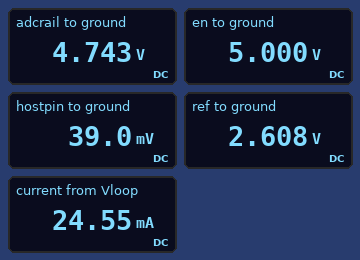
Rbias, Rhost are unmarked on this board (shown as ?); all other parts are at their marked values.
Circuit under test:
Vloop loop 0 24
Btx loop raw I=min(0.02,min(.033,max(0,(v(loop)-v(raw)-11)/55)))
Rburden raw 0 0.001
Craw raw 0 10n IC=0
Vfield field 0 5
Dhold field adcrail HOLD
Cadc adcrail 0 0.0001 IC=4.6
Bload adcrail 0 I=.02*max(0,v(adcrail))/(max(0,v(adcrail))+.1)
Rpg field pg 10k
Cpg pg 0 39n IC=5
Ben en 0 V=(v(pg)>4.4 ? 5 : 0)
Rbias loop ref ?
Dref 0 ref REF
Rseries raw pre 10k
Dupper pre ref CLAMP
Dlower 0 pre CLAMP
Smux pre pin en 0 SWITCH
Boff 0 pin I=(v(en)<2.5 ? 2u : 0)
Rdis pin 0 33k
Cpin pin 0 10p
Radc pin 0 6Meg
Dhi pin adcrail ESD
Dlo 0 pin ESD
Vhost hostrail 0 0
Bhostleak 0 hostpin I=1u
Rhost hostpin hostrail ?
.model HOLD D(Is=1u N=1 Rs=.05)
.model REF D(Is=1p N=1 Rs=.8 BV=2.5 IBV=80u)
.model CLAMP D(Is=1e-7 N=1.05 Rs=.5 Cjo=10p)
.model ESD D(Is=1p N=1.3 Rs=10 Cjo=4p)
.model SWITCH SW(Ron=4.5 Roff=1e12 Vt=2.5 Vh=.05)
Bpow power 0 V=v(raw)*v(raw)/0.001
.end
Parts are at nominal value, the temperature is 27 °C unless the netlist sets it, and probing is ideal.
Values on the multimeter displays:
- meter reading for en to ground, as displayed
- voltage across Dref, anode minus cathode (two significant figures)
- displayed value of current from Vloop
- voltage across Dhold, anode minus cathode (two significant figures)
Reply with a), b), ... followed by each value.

a) 5.000 V
b) -2.6 V
c) 24.55 mA
d) 260 mV
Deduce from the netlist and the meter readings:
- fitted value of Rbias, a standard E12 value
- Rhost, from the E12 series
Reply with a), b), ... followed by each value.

a) 4.7 kΩ
b) 39 kΩ
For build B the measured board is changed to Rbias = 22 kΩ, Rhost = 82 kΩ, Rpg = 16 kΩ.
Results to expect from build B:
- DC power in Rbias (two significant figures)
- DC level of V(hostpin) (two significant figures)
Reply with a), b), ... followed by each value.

a) 21 mW
b) 82 mV
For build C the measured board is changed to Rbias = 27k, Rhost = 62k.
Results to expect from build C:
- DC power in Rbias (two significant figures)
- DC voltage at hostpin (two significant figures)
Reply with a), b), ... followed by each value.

a) 17 mW
b) 62 mV
